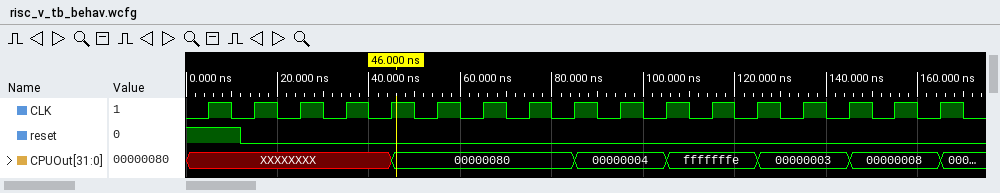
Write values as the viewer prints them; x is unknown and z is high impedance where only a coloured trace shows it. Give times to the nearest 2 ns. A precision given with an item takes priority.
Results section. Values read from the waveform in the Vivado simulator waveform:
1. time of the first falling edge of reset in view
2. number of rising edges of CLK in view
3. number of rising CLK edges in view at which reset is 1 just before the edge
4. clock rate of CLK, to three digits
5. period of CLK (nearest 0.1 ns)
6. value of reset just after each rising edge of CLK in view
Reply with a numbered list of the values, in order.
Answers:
1. 12 ns
2. 17
3. 1
4. 100 MHz
5. 10 ns
6. 1 0 0 0 0 0 0 0 0 0 0 0 0 0 0 0 0
